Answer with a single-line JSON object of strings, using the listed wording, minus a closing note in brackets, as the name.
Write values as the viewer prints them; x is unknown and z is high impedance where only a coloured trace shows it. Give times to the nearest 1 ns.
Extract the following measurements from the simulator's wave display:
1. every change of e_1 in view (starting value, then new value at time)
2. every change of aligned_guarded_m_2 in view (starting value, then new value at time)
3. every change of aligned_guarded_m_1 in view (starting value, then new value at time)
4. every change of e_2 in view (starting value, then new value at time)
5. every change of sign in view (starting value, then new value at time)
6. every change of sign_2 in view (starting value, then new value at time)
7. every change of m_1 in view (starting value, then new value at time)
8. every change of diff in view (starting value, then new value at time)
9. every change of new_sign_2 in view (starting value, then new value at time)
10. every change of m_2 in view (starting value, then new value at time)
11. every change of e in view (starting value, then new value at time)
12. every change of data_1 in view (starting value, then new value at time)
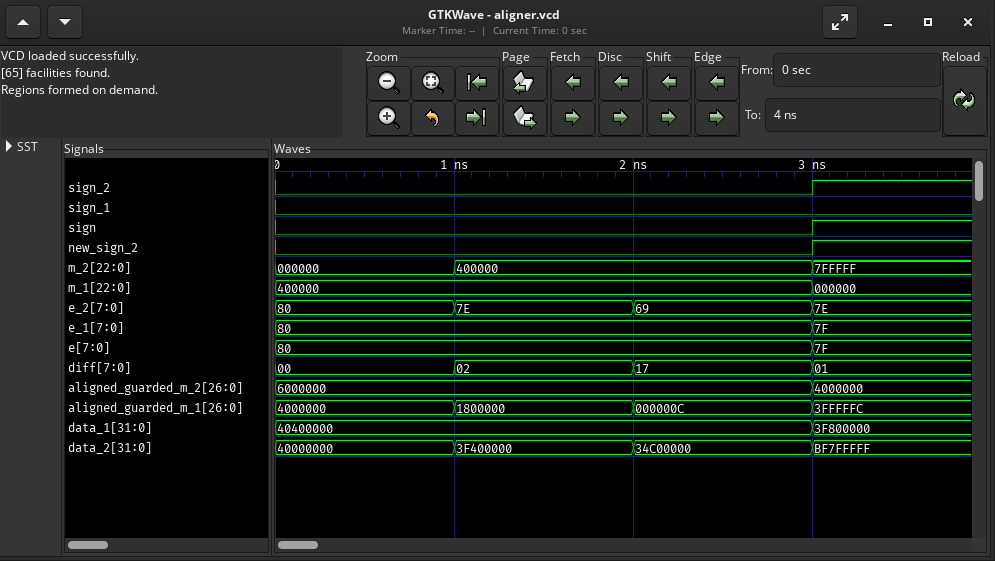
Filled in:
{"every change of e_1 in view": "80, 7F at 3 ns", "every change of aligned_guarded_m_2 in view": "6000000, 4000000 at 3 ns", "every change of aligned_guarded_m_1 in view": "4000000, 1800000 at 1 ns, 000000C at 2 ns, 3FFFFFC at 3 ns", "every change of e_2 in view": "80, 7E at 1 ns, 69 at 2 ns, 7E at 3 ns", "every change of sign in view": "0, 1 at 3 ns", "every change of sign_2 in view": "0, 1 at 3 ns", "every change of m_1 in view": "400000, 000000 at 3 ns", "every change of diff in view": "00, 02 at 1 ns, 17 at 2 ns, 01 at 3 ns", "every change of new_sign_2 in view": "0, 1 at 3 ns", "every change of m_2 in view": "000000, 400000 at 1 ns, 7FFFFF at 3 ns", "every change of e in view": "80, 7F at 3 ns", "every change of data_1 in view": "40400000, 3F800000 at 3 ns"}
